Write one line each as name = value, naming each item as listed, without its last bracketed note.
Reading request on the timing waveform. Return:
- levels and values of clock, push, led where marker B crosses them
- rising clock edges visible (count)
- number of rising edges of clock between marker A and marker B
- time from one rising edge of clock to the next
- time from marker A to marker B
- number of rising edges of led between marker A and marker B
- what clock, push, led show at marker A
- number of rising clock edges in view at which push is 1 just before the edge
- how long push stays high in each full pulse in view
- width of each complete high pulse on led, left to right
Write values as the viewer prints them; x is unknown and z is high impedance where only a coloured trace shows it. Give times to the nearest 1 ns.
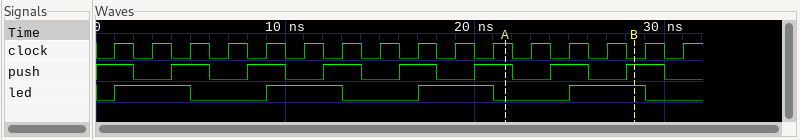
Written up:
levels and values of clock, push, led where marker B crosses them = clock=0, push=1, led=1
rising clock edges visible = 16
number of rising edges of clock between marker A and marker B = 3
time from one rising edge of clock to the next = 2 ns
time from marker A to marker B = 7 ns
number of rising edges of led between marker A and marker B = 1
what clock, push, led show at marker A = clock=1, push=1, led=0
number of rising clock edges in view at which push is 1 just before the edge = 8
how long push stays high in each full pulse in view = 2 ns, 2 ns, 2 ns, 2 ns, 2 ns, 2 ns, 2 ns
width of each complete high pulse on led, left to right = 4 ns, 4 ns, 4 ns, 4 ns
